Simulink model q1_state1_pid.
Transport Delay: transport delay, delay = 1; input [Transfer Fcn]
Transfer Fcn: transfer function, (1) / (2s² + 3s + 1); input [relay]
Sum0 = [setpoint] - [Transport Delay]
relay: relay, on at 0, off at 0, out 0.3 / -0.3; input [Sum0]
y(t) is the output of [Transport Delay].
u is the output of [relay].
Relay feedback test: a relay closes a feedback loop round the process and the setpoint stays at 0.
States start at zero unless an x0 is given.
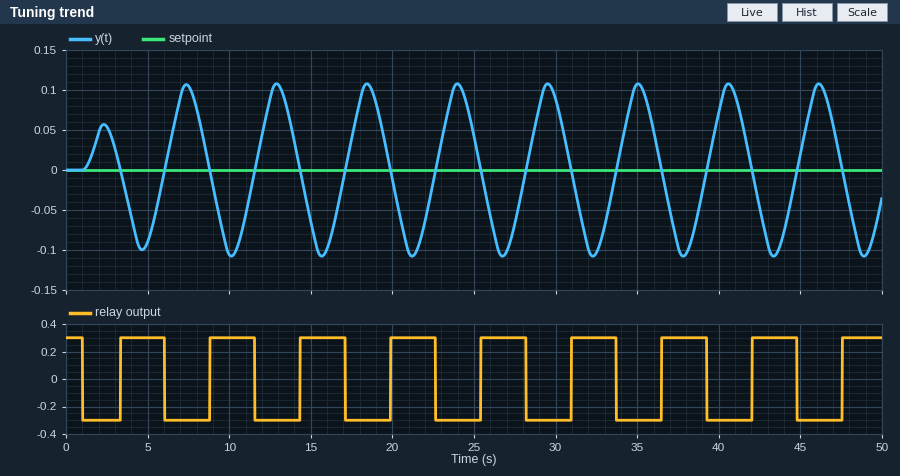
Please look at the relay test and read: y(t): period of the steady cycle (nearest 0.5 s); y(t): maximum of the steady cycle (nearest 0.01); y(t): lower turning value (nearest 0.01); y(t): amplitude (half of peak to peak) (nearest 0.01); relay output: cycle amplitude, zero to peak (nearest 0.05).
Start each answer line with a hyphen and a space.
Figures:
- 5.5 s
- 0.11
- -0.11
- 0.11
- 0.30
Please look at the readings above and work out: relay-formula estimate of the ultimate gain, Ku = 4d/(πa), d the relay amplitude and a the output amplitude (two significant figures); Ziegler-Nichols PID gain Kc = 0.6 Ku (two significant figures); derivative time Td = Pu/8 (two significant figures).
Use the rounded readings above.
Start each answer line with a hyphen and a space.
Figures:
- 3.5
- 2.1
- 0.69 s
